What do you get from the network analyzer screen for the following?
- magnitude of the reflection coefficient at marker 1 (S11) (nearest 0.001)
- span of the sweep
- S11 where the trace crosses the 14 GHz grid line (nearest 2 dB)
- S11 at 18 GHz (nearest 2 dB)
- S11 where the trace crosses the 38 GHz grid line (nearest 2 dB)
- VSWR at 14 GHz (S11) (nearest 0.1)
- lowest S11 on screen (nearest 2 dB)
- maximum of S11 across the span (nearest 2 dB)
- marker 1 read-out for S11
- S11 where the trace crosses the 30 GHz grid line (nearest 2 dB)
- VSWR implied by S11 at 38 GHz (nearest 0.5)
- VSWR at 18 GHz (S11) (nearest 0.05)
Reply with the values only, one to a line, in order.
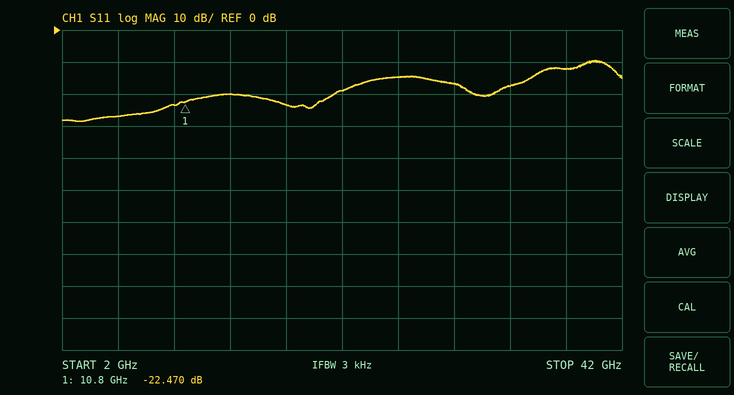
0.075
40 GHz
-20 dB
-24 dB
-12 dB
1.2
-28 dB
-10 dB
-22.470 dB
-16 dB
1.5
1.15
